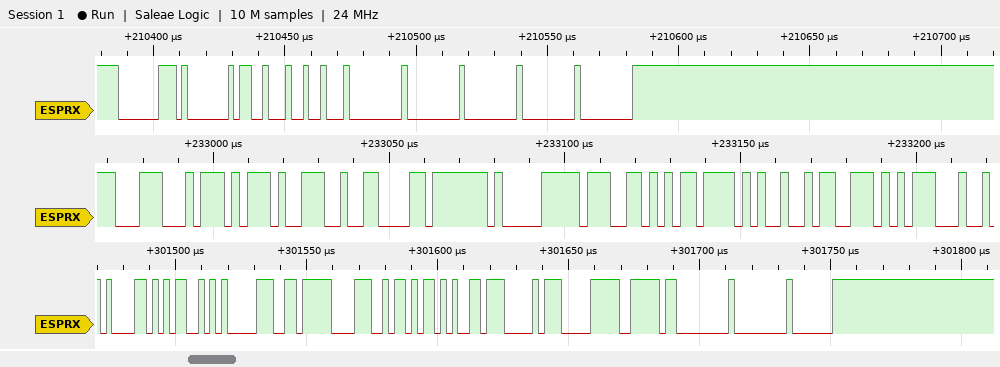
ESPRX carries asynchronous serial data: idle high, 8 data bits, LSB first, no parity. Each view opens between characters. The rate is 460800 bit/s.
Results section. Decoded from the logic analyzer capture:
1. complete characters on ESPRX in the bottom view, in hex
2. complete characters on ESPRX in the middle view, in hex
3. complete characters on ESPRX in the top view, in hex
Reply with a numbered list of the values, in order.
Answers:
1. 61, 4D, C1, F6, 38, 6B, D9, D0, F0, BE, 00, 00, C0
2. 1C, D7, 39, 86, 7F, F0, 67, ED, 25, 73, 1D
3. C0, 01, 13, 12, 00, 00, 00, 00, 00
